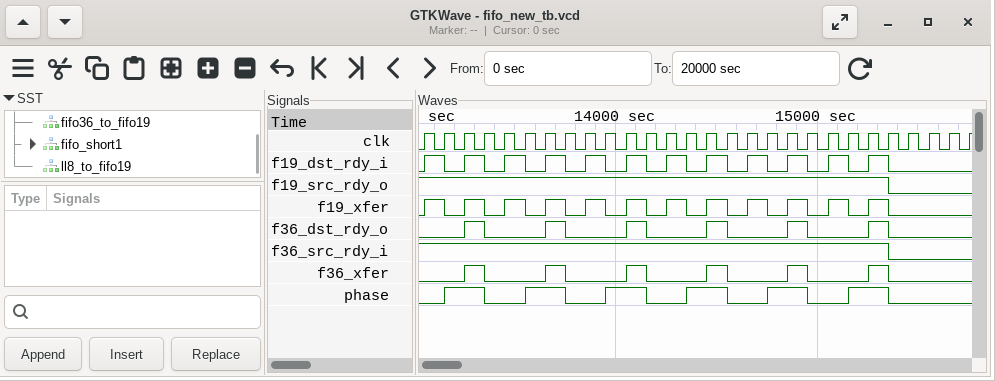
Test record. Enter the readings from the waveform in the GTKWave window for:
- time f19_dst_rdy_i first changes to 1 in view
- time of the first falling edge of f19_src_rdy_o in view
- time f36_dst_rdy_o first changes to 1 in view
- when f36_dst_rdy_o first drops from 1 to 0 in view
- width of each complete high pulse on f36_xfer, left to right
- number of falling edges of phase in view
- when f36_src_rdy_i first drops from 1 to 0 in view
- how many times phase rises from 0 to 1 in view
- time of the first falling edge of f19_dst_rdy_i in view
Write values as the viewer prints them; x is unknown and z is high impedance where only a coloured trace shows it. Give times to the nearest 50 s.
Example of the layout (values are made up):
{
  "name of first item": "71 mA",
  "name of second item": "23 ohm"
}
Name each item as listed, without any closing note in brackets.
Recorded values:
{
  "time f19_dst_rdy_i first changes to 1 in view": "13050 s",
  "time of the first falling edge of f19_src_rdy_o in view": "15350 s",
  "time f36_dst_rdy_o first changes to 1 in view": "13250 s",
  "when f36_dst_rdy_o first drops from 1 to 0 in view": "13350 s",
  "width of each complete high pulse on f36_xfer, left to right": "100 s, 100 s, 100 s, 100 s, 100 s, 100 s",
  "number of falling edges of phase in view": "6",
  "when f36_src_rdy_i first drops from 1 to 0 in view": "15350 s",
  "how many times phase rises from 0 to 1 in view": "6",
  "time of the first falling edge of f19_dst_rdy_i in view": "13150 s"
}
